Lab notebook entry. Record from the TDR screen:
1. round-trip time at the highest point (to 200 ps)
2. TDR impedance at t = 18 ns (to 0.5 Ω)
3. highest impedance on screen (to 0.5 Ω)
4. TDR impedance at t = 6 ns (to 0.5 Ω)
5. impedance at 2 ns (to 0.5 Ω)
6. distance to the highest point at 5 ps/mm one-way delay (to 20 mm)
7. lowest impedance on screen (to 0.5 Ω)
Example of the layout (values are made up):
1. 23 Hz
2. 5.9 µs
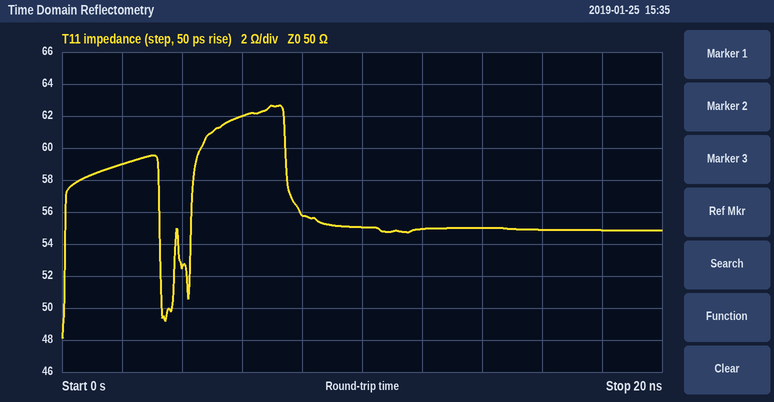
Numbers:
1. 7.2 ns
2. 55.0 Ω
3. 62.5 Ω
4. 62.0 Ω
5. 59.0 Ω
6. 720 mm
7. 48.0 Ω
